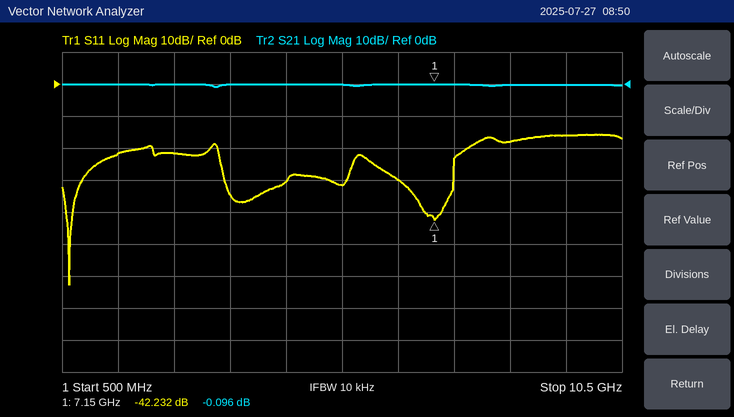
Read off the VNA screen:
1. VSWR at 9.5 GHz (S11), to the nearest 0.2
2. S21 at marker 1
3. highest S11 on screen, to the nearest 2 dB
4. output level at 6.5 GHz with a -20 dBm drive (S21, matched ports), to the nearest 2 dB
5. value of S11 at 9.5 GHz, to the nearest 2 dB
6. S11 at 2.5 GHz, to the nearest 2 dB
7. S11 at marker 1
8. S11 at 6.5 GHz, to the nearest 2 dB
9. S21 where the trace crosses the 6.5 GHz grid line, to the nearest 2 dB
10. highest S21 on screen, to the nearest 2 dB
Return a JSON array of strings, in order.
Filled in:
["1.4", "-0.096 dB", "-16 dB", "-20 dBm", "-16 dB", "-22 dB", "-42.232 dB", "-30 dB", "0 dB", "0 dB"]
